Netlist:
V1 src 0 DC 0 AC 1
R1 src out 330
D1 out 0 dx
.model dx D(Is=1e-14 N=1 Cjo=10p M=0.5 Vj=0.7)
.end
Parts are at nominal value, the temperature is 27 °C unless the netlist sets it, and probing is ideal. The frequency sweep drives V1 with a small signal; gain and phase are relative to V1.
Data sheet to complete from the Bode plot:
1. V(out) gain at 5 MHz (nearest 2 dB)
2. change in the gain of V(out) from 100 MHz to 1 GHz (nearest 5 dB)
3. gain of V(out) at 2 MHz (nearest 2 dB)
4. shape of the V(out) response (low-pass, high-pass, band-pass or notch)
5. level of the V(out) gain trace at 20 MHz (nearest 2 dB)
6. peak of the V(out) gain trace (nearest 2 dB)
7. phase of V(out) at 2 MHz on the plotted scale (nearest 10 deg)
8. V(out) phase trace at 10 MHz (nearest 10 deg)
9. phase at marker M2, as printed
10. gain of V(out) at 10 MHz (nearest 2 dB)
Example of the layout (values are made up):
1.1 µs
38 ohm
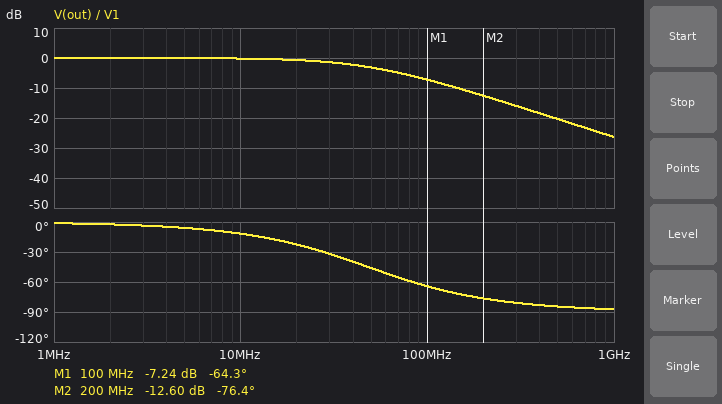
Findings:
0 dB
-20 dB
0 dB
low-pass
0 dB
0 dB
0 deg
-10 deg
-76.4 deg
0 dB
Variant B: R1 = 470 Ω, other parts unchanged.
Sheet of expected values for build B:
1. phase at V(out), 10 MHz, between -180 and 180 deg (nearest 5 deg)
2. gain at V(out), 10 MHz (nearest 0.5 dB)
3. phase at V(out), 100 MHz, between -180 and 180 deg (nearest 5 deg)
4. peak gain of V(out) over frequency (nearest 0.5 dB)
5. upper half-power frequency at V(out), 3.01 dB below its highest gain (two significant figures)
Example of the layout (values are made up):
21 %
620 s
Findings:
-15 deg
-0.5 dB
-70 deg
0 dB
34 MHz
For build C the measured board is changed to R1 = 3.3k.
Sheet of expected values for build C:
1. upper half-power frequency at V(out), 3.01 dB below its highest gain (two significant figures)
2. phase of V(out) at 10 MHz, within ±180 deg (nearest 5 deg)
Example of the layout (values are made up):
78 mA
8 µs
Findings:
4.8 MHz
-65 deg
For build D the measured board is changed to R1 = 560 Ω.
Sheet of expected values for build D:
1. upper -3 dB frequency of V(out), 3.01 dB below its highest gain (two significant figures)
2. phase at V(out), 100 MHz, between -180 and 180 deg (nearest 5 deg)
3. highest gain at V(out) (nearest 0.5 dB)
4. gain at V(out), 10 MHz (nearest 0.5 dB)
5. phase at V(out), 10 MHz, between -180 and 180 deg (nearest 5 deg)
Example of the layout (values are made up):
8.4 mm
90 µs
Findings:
28 MHz
-75 deg
0 dB
-0.5 dB
-20 deg
